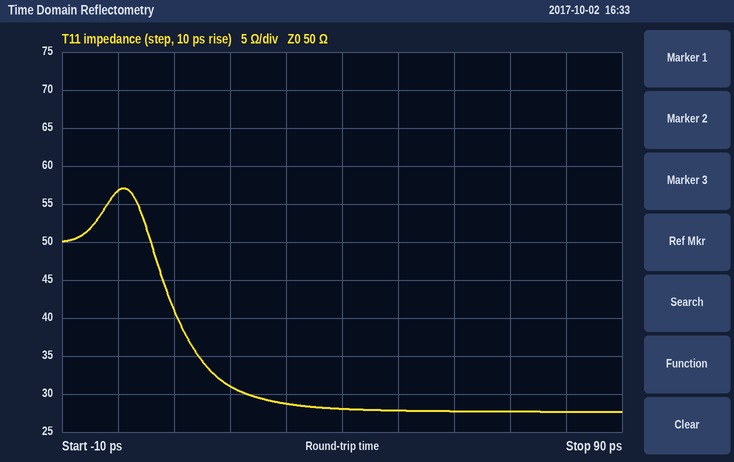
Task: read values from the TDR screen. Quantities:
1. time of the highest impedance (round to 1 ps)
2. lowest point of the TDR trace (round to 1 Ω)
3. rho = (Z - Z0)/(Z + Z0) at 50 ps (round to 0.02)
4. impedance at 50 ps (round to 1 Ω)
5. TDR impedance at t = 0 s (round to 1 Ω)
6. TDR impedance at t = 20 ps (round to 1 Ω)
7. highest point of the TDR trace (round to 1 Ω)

1 ps
28 Ω
-0.28
28 Ω
57 Ω
31 Ω
57 Ω
